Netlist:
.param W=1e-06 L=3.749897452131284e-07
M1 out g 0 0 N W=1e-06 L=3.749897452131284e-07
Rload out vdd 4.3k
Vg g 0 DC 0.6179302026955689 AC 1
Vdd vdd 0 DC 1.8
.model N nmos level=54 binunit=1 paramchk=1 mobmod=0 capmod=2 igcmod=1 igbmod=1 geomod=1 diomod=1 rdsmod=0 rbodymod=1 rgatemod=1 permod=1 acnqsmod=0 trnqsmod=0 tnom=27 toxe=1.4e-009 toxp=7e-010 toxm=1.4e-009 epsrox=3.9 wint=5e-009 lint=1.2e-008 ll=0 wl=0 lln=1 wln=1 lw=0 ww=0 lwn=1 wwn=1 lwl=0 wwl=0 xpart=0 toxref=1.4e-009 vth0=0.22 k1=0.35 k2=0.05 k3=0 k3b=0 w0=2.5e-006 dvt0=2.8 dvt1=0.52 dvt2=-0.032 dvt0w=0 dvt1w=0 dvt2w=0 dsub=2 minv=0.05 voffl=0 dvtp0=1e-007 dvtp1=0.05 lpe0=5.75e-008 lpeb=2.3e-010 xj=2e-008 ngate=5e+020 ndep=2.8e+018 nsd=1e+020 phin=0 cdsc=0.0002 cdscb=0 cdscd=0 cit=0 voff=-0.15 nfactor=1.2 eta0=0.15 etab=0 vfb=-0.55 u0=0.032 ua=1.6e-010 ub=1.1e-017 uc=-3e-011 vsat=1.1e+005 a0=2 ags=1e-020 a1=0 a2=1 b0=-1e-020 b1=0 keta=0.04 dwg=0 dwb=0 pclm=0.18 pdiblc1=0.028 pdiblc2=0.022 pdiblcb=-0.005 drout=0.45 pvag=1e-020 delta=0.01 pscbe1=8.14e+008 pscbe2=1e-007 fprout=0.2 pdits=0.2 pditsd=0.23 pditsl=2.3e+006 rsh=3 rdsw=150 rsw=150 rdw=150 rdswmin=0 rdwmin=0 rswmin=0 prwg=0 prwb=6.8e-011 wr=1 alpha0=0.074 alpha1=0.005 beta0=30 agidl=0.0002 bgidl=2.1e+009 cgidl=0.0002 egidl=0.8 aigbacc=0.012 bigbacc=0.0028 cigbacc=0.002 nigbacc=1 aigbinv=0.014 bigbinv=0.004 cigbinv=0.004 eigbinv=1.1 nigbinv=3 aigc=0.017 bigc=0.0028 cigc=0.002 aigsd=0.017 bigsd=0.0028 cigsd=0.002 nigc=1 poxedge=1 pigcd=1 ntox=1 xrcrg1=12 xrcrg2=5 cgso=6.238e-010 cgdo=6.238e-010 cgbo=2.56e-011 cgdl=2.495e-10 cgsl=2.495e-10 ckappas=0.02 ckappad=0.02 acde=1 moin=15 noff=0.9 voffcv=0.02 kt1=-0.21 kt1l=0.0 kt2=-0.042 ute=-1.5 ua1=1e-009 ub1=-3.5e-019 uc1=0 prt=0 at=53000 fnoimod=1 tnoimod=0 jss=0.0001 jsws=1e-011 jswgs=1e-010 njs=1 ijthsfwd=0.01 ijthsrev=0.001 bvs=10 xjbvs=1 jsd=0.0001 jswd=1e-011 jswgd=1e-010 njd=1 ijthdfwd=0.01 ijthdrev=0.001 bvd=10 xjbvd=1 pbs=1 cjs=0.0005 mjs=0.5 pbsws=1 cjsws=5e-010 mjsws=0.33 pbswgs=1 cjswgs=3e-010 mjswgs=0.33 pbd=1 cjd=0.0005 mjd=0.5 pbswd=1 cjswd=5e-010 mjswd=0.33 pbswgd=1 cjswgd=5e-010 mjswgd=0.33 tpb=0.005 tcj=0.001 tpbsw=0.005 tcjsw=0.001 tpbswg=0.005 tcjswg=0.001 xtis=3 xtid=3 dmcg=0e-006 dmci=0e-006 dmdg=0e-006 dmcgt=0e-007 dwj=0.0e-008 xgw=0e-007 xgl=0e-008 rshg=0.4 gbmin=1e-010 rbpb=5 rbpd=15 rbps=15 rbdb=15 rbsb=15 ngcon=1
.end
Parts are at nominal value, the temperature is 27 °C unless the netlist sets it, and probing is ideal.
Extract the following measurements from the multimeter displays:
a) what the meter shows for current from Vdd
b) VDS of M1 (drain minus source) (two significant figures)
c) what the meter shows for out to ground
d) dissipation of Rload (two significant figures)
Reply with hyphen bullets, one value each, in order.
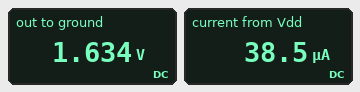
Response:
- 38.5 µA
- 1.6 V
- 1.634 V
- 6.4 µW
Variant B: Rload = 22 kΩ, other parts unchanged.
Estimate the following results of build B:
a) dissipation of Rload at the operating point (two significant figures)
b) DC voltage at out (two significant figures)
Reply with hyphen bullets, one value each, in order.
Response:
- 27 µW
- 1.0 V
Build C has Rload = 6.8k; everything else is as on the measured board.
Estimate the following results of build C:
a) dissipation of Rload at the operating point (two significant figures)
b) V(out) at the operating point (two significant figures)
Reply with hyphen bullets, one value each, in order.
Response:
- 9.8 µW
- 1.5 V
